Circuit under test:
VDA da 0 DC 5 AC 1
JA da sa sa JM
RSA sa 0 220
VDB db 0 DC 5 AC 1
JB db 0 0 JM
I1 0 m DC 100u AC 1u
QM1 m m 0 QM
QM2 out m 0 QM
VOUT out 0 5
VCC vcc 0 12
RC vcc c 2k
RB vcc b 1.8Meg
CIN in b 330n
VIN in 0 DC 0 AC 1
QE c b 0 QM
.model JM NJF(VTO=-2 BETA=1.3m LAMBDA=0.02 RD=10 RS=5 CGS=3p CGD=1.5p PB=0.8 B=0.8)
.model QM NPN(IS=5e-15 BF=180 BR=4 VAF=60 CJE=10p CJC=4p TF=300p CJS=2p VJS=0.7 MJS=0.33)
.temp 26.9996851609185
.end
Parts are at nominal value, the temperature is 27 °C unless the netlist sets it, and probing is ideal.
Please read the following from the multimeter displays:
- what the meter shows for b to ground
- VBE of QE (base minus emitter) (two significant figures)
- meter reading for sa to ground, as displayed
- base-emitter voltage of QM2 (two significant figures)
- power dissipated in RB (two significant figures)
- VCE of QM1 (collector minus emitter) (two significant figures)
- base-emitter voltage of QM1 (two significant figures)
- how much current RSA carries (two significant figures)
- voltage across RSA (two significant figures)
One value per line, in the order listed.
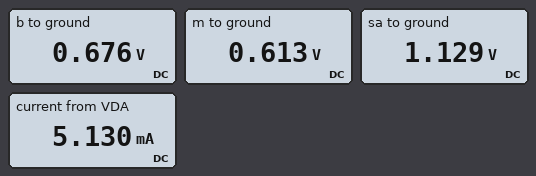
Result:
0.676 V
680 mV
1.129 V
610 mV
71 µW
610 mV
610 mV
5.1 mA
1.1 V
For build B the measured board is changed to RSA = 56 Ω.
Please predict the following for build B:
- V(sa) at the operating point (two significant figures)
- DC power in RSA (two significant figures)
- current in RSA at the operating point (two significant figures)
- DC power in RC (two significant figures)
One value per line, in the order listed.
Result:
290 mV
1.5 mW
5.2 mA
3.4 mW
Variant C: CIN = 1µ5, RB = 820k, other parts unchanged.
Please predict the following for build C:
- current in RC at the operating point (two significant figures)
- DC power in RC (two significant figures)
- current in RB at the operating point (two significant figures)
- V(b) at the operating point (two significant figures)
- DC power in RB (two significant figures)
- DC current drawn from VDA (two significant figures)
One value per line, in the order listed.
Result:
2.7 mA
15 mW
14 µA
700 mV
160 µW
5.1 mA
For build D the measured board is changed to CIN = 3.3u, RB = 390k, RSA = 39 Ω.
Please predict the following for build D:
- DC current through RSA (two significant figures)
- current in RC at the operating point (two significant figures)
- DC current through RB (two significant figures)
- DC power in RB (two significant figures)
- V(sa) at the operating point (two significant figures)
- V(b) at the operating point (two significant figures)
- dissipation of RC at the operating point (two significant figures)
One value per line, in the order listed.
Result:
5.2 mA
5.3 mA
29 µA
330 µW
200 mV
720 mV
56 mW
